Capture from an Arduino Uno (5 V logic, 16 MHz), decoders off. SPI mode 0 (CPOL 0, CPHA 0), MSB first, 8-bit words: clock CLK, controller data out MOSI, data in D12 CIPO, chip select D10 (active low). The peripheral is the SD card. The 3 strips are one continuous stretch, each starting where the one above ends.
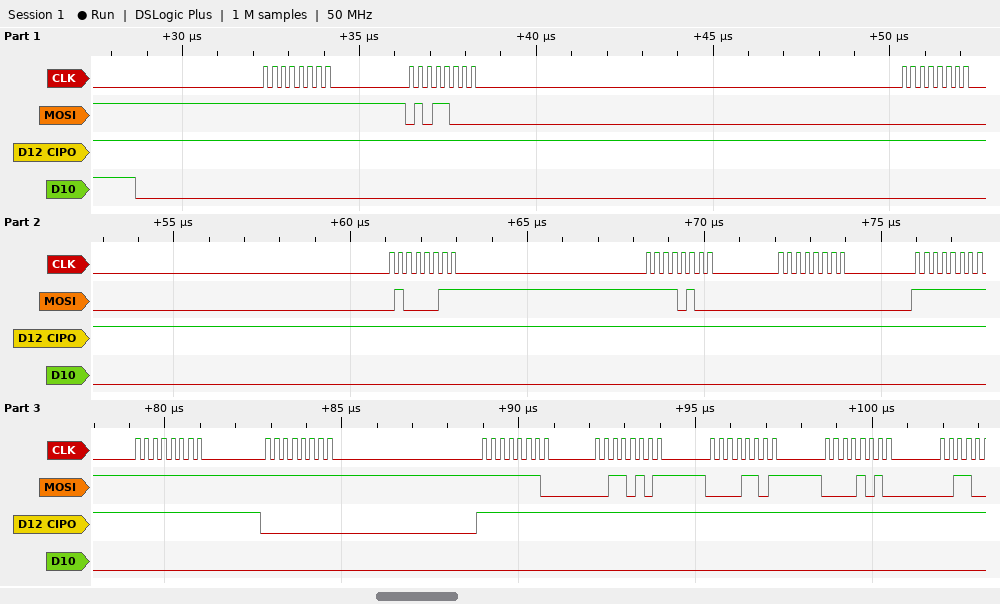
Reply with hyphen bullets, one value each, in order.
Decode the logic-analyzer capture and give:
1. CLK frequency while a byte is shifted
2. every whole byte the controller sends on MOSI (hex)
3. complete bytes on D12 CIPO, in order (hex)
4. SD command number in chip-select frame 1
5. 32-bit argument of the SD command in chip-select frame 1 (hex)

- 4 MHz
- FF 58 00 43 F4 00 FF FF FF FE 35 0D 0A
- FF FF FF FF FF FF FF FF 00 FF FF FF FF
- CMD24
- 0x0043F400
